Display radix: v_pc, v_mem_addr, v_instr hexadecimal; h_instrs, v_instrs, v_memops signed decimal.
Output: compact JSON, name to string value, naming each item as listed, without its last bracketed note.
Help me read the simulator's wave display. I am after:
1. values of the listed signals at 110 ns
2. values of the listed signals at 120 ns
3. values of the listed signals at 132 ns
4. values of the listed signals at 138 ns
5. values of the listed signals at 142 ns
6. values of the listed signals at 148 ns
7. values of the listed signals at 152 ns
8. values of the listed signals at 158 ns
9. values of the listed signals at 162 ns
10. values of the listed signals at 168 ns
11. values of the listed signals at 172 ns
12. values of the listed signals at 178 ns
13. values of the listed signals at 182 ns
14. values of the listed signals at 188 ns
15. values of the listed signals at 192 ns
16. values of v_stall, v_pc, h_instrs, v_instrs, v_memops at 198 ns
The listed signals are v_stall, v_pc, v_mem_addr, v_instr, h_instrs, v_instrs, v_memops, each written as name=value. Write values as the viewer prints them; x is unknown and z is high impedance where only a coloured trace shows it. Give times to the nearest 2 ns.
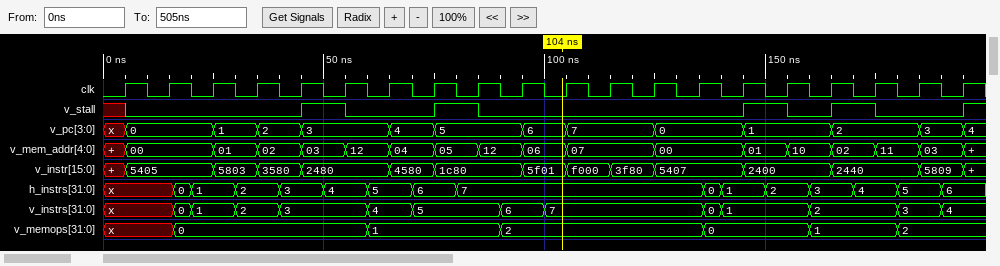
{"values of the listed signals at 110 ns": "v_stall=0, v_pc=7, v_mem_addr=07, v_instr=f000, h_instrs=7, v_instrs=7, v_memops=2", "values of the listed signals at 120 ns": "v_stall=0, v_pc=7, v_mem_addr=07, v_instr=3f80, h_instrs=7, v_instrs=7, v_memops=2", "values of the listed signals at 132 ns": "v_stall=0, v_pc=0, v_mem_addr=00, v_instr=5407, h_instrs=7, v_instrs=7, v_memops=2", "values of the listed signals at 138 ns": "v_stall=0, v_pc=0, v_mem_addr=00, v_instr=5407, h_instrs=0, v_instrs=0, v_memops=0", "values of the listed signals at 142 ns": "v_stall=0, v_pc=0, v_mem_addr=00, v_instr=5407, h_instrs=1, v_instrs=1, v_memops=0", "values of the listed signals at 148 ns": "v_stall=1, v_pc=1, v_mem_addr=01, v_instr=2400, h_instrs=1, v_instrs=1, v_memops=0", "values of the listed signals at 152 ns": "v_stall=1, v_pc=1, v_mem_addr=01, v_instr=2400, h_instrs=2, v_instrs=1, v_memops=0", "values of the listed signals at 158 ns": "v_stall=0, v_pc=1, v_mem_addr=10, v_instr=2400, h_instrs=2, v_instrs=1, v_memops=0", "values of the listed signals at 162 ns": "v_stall=0, v_pc=1, v_mem_addr=10, v_instr=2400, h_instrs=3, v_instrs=2, v_memops=1", "values of the listed signals at 168 ns": "v_stall=1, v_pc=2, v_mem_addr=02, v_instr=2440, h_instrs=3, v_instrs=2, v_memops=1", "values of the listed signals at 172 ns": "v_stall=1, v_pc=2, v_mem_addr=02, v_instr=2440, h_instrs=4, v_instrs=2, v_memops=1", "values of the listed signals at 178 ns": "v_stall=0, v_pc=2, v_mem_addr=11, v_instr=2440, h_instrs=4, v_instrs=2, v_memops=1", "values of the listed signals at 182 ns": "v_stall=0, v_pc=2, v_mem_addr=11, v_instr=2440, h_instrs=5, v_instrs=3, v_memops=2", "values of the listed signals at 188 ns": "v_stall=0, v_pc=3, v_mem_addr=03, v_instr=5809, h_instrs=5, v_instrs=3, v_memops=2", "values of the listed signals at 192 ns": "v_stall=0, v_pc=3, v_mem_addr=03, v_instr=5809, h_instrs=6, v_instrs=4, v_memops=2", "values of v_stall, v_pc, h_instrs, v_instrs, v_memops at 198 ns": "v_stall=1, v_pc=4, h_instrs=6, v_instrs=4, v_memops=2"}
